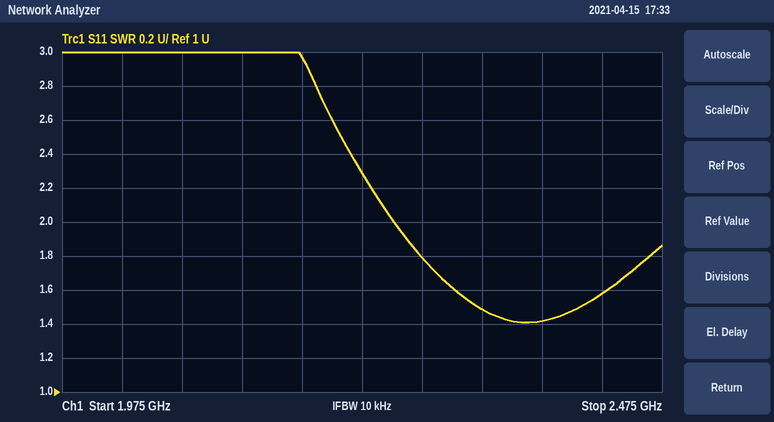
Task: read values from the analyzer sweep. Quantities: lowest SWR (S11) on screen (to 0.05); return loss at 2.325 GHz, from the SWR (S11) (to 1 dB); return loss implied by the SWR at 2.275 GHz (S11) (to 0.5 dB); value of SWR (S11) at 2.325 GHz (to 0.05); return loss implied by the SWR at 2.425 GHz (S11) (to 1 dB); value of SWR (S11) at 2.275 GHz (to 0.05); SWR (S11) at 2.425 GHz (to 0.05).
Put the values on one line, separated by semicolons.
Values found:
1.40; 14 dB; 11.0 dB; 1.50; 13 dB; 1.80; 1.60
